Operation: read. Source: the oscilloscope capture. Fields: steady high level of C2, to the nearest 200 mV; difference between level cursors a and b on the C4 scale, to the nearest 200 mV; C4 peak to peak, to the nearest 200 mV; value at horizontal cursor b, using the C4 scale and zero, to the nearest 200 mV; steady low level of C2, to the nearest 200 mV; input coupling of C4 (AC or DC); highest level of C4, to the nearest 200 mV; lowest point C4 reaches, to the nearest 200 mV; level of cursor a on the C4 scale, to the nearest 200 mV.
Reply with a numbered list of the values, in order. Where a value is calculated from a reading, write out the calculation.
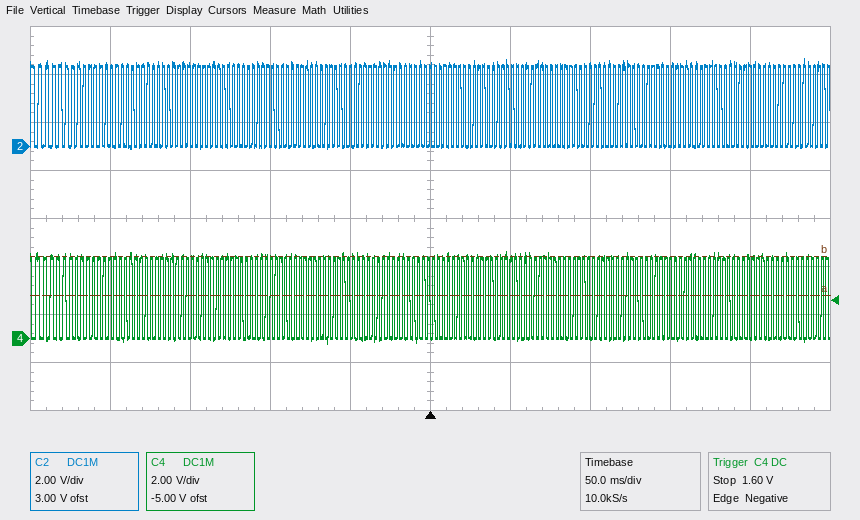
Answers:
1. 3.4 V
2. 1.6 V
3. 3.6 V − (-200 mV) = 3.8 V
4. 3.4 V
5. 0.0 V
6. DC
7. 3.6 V
8. -200 mV
9. 1.8 V
